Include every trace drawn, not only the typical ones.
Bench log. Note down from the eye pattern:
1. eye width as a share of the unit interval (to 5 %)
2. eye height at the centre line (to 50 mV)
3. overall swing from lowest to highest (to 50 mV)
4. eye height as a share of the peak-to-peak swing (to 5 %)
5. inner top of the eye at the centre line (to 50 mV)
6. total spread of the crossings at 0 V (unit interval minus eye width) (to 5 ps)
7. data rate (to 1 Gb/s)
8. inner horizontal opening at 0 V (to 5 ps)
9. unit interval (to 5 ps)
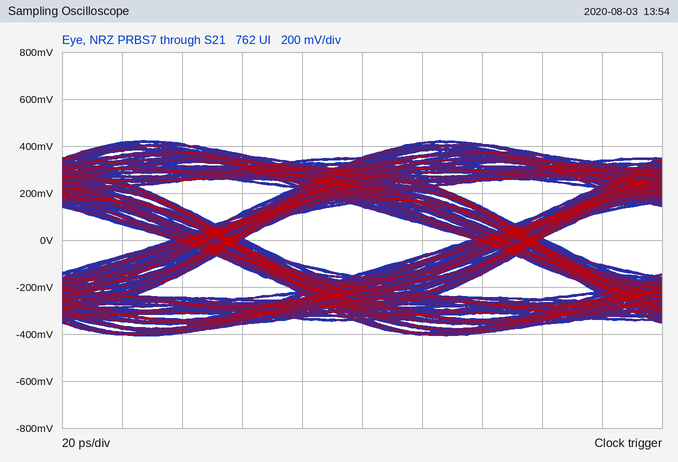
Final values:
75 %
300 mV
850 mV
35 %
150 mV
25 ps
10 Gb/s
75 ps
100 ps
